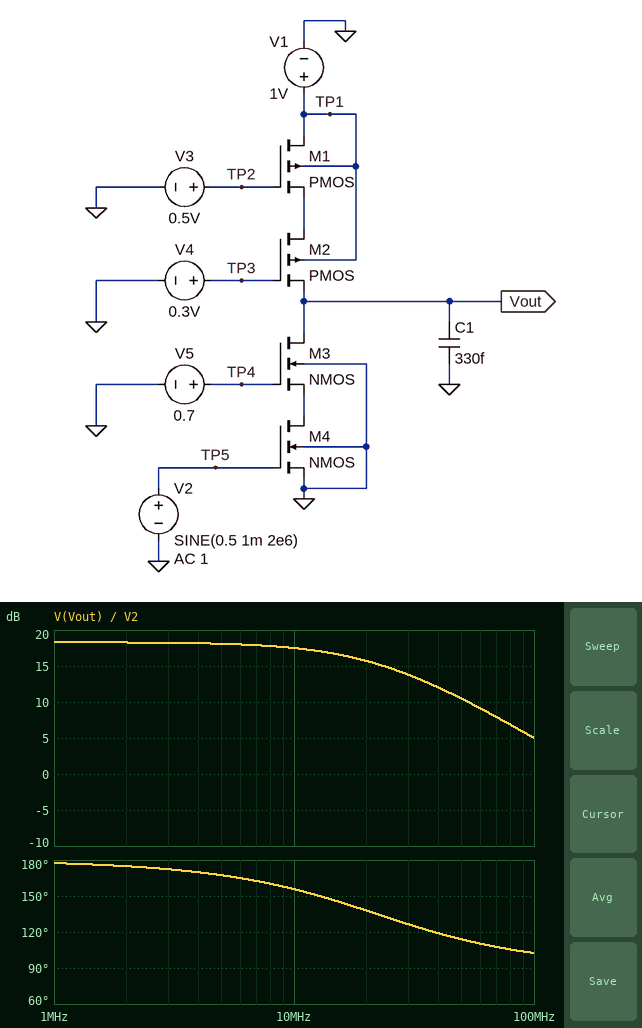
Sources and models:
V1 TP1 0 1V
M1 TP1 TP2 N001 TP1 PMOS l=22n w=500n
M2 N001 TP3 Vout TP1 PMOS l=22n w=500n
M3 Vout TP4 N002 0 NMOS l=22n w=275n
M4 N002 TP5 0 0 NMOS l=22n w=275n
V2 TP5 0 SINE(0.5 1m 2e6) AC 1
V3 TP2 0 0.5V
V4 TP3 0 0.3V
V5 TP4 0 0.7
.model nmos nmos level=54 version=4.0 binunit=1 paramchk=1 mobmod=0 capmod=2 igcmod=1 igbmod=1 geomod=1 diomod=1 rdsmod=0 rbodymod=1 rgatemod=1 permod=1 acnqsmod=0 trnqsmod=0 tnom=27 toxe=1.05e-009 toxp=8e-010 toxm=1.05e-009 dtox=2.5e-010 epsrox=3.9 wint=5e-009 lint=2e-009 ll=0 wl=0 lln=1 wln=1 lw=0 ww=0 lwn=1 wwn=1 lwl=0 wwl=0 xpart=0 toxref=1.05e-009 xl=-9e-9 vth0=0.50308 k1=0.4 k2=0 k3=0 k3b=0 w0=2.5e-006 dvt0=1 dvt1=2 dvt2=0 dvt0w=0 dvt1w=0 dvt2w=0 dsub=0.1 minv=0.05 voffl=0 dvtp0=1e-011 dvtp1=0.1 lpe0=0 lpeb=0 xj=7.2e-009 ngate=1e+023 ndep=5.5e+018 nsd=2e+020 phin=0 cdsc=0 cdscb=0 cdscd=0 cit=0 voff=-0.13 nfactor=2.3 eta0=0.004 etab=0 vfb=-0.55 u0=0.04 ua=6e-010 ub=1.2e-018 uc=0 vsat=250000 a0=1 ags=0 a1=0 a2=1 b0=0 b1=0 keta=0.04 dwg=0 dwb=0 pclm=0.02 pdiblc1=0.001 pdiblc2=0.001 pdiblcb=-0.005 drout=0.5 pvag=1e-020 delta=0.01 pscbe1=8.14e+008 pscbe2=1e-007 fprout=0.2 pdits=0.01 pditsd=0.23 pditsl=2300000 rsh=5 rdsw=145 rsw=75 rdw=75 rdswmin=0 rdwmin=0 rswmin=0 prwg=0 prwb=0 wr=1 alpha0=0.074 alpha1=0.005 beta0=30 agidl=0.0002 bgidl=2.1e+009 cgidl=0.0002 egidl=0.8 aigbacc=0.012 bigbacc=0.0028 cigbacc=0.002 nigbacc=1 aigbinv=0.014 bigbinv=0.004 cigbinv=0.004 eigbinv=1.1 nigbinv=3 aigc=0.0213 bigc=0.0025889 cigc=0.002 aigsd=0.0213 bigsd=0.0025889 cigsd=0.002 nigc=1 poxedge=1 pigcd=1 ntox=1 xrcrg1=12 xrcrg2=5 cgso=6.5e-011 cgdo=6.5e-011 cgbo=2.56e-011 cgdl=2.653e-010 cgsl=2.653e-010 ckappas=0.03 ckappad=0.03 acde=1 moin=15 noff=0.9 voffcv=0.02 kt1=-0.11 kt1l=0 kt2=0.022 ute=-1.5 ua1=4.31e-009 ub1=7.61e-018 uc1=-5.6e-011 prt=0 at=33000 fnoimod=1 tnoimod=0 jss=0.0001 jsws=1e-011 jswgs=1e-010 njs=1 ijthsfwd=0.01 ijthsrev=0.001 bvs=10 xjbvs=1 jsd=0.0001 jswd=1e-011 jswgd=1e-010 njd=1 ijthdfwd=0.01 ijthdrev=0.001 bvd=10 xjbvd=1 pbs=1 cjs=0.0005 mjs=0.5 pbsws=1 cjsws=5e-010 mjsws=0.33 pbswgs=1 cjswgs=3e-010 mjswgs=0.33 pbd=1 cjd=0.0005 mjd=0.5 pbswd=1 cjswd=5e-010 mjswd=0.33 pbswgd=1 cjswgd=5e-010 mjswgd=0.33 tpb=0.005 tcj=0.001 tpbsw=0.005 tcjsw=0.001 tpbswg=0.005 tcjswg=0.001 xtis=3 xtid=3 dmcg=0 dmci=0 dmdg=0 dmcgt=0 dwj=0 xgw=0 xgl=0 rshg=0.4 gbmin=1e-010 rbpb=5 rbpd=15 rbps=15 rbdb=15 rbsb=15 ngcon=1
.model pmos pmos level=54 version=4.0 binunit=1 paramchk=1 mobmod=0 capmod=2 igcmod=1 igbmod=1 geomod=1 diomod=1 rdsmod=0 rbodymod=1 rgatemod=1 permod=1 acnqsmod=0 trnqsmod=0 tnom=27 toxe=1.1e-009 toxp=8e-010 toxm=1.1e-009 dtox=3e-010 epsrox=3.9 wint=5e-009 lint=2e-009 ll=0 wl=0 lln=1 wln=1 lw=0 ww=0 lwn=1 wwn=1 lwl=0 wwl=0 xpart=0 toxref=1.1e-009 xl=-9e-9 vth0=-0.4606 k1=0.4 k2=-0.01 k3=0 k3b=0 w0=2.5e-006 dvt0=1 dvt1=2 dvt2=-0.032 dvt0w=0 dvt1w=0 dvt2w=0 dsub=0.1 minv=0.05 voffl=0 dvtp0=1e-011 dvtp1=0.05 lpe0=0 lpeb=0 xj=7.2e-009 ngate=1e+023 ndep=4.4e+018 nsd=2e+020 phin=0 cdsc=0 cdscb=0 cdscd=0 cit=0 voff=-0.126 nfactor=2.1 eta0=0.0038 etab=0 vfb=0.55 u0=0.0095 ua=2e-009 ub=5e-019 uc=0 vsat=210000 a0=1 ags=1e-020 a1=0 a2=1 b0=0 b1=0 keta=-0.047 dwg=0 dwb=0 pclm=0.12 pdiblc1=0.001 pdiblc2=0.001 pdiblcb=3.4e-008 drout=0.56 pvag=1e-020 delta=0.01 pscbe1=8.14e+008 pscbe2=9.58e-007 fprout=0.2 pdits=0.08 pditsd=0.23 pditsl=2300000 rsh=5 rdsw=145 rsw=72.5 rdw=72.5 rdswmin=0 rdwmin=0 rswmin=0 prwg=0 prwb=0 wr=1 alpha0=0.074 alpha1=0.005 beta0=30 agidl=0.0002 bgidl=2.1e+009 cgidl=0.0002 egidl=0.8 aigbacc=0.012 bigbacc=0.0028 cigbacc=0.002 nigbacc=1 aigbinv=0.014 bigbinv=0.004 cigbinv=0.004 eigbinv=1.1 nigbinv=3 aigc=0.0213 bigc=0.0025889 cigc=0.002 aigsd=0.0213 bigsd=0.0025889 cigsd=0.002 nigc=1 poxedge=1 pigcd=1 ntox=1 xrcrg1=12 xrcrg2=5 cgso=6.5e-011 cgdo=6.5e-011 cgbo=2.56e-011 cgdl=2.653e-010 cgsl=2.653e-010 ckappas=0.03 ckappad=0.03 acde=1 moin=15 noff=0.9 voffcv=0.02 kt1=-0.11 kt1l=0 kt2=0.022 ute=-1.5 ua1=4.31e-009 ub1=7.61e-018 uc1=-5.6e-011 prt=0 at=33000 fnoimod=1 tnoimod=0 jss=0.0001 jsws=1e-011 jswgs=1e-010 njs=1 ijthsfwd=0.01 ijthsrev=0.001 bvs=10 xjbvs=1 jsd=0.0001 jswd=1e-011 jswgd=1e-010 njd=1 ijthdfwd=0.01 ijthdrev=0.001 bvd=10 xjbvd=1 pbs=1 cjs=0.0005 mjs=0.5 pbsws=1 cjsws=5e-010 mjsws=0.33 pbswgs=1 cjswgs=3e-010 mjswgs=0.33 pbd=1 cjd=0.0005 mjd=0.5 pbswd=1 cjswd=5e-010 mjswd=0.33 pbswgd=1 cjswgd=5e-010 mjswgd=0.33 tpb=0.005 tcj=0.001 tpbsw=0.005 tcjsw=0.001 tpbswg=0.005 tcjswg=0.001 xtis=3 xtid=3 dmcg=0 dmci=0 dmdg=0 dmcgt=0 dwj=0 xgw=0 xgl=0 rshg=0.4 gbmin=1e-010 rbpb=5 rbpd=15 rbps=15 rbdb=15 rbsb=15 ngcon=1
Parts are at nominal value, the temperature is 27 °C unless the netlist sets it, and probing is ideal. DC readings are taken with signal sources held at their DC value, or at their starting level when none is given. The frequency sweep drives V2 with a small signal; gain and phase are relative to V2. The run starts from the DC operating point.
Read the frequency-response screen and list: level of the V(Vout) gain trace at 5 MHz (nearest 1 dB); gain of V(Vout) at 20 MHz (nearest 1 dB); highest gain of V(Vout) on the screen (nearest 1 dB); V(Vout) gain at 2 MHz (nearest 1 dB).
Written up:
18 dB
16 dB
18 dB
18 dB
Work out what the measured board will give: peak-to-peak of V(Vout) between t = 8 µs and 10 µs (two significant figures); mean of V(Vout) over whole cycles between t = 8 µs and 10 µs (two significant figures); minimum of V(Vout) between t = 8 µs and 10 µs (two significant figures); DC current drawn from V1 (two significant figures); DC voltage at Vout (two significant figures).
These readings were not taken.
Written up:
16 mV
520 mV
510 mV
38 µA
520 mV
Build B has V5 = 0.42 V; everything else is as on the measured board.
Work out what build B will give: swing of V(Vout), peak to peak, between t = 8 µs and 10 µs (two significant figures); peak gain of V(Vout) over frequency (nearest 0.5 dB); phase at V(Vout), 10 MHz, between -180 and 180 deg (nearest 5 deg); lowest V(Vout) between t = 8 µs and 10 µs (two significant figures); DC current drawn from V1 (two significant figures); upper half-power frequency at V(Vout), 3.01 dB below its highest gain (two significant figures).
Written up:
3.8 mV
5.5 dB
170 deg
840 mV
24 µA
57 MHz
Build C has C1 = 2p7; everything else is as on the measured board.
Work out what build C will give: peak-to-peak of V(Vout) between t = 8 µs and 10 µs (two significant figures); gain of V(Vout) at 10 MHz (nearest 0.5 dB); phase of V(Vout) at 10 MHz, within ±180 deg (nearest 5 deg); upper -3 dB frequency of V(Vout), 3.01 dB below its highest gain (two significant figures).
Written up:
13 mV
6.5 dB
105 deg
2.7 MHz
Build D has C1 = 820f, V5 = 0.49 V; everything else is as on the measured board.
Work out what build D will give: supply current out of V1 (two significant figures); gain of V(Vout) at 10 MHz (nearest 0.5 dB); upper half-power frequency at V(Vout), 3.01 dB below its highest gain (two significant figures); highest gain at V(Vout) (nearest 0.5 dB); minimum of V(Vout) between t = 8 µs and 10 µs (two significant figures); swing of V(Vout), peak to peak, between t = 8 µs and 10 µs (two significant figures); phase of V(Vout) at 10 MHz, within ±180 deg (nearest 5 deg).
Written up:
28 µA
9.0 dB
17 MHz
10.5 dB
790 mV
6.5 mV
150 deg
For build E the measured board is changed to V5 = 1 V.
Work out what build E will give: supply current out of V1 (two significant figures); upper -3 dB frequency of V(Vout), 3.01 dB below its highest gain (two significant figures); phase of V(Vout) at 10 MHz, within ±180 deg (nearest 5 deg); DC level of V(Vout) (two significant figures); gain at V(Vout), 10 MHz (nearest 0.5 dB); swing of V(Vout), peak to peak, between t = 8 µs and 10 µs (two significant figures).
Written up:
44 µA
65 MHz
170 deg
290 mV
10.0 dB
6.5 mV
